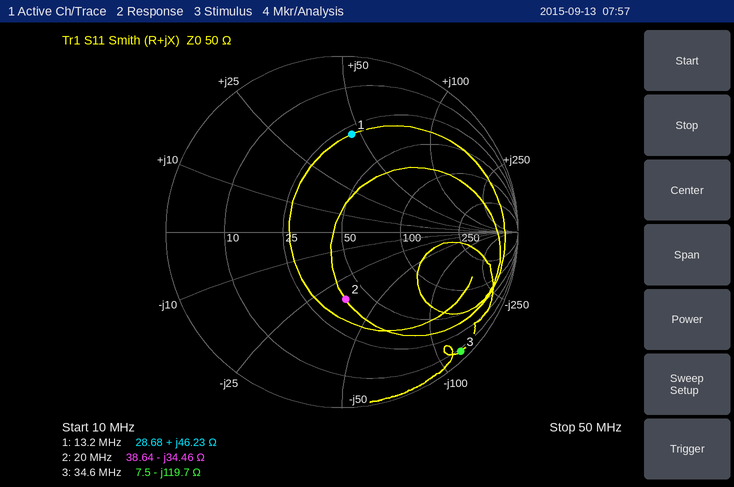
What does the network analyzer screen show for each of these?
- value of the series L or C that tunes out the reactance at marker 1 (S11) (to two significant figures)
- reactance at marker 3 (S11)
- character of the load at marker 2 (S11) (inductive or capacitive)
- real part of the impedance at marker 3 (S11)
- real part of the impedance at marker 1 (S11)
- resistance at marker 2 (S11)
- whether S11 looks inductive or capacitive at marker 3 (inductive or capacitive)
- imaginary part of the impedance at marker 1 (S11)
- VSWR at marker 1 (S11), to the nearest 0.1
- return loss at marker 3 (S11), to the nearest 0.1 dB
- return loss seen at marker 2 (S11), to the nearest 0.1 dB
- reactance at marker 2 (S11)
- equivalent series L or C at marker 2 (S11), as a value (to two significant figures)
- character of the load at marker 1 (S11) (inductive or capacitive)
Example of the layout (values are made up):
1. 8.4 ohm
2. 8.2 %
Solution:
1. 260 pF
2. -119.7 Ω
3. capacitive
4. 7.5 Ω
5. 28.68 Ω
6. 38.64 Ω
7. capacitive
8. +46.23 Ω
9. 3.5
10. 0.4 dB
11. 8.4 dB
12. -34.46 Ω
13. 230 pF
14. inductive
